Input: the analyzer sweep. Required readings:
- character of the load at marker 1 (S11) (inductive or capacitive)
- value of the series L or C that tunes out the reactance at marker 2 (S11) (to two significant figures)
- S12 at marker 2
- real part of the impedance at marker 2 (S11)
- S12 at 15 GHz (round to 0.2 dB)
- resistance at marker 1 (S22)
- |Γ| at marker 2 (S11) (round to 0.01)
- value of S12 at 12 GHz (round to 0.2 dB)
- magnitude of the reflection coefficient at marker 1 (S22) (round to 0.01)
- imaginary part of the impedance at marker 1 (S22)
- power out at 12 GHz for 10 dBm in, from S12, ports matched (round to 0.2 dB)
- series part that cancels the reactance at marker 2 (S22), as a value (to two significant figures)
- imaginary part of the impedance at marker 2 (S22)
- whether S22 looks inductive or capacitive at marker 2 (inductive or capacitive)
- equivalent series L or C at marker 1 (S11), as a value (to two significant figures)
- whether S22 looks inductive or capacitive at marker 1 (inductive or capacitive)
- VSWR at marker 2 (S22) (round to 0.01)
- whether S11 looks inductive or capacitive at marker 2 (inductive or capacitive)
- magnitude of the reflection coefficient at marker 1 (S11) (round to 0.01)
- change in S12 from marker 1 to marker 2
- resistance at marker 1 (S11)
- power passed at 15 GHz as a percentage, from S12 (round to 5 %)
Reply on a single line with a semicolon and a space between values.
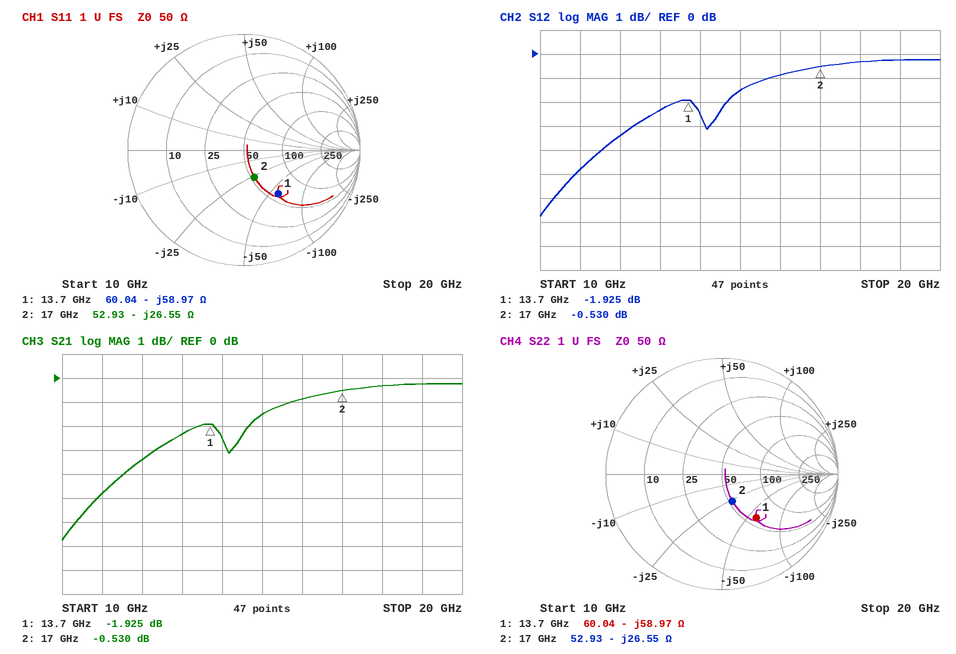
capacitive; 250 pH; -0.530 dB; 52.93 Ω; -1.6 dB; 60.04 Ω; 0.25; -3.4 dB; 0.48; -58.97 Ω; 6.6 dBm; 250 pH; -26.55 Ω; capacitive; 200 fF; capacitive; 1.67; capacitive; 0.48; 1.395 dB; 60.04 Ω; 70 %
